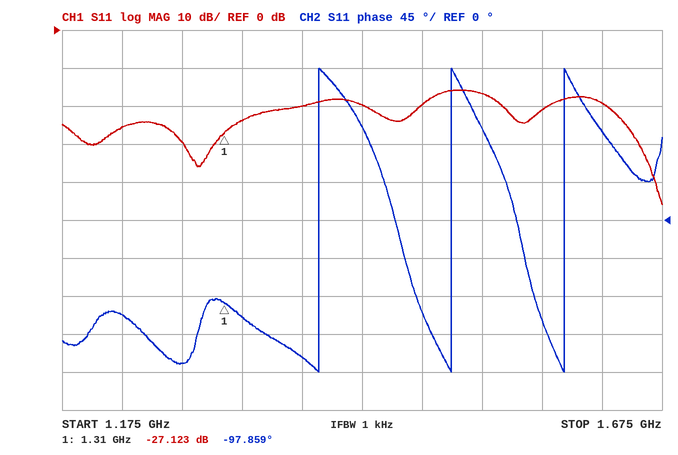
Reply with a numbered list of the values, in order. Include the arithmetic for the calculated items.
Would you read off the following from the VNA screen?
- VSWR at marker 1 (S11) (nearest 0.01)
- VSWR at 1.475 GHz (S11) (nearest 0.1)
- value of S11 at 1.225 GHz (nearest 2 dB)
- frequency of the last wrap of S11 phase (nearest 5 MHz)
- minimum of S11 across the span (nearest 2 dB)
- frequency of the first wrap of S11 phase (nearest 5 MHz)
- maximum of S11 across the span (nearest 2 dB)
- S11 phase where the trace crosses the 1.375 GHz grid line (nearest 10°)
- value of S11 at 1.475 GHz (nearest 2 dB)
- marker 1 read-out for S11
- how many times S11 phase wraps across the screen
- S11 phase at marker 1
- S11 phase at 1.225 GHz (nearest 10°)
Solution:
1. (1 + 0.0440)/(1 − 0.0440) ≈ 1.09
2. |Γ| = 10^(-20/20) = 0.1000; VSWR = (1 + 0.1000)/(1 − 0.1000) ≈ 1.2
3. -26 dB
4. 1.595 GHz
5. -46 dB
6. 1.390 GHz
7. -16 dB
8. -160°
9. -20 dB
10. -27.123 dB
11. 3
12. -97.859°
13. -110°
